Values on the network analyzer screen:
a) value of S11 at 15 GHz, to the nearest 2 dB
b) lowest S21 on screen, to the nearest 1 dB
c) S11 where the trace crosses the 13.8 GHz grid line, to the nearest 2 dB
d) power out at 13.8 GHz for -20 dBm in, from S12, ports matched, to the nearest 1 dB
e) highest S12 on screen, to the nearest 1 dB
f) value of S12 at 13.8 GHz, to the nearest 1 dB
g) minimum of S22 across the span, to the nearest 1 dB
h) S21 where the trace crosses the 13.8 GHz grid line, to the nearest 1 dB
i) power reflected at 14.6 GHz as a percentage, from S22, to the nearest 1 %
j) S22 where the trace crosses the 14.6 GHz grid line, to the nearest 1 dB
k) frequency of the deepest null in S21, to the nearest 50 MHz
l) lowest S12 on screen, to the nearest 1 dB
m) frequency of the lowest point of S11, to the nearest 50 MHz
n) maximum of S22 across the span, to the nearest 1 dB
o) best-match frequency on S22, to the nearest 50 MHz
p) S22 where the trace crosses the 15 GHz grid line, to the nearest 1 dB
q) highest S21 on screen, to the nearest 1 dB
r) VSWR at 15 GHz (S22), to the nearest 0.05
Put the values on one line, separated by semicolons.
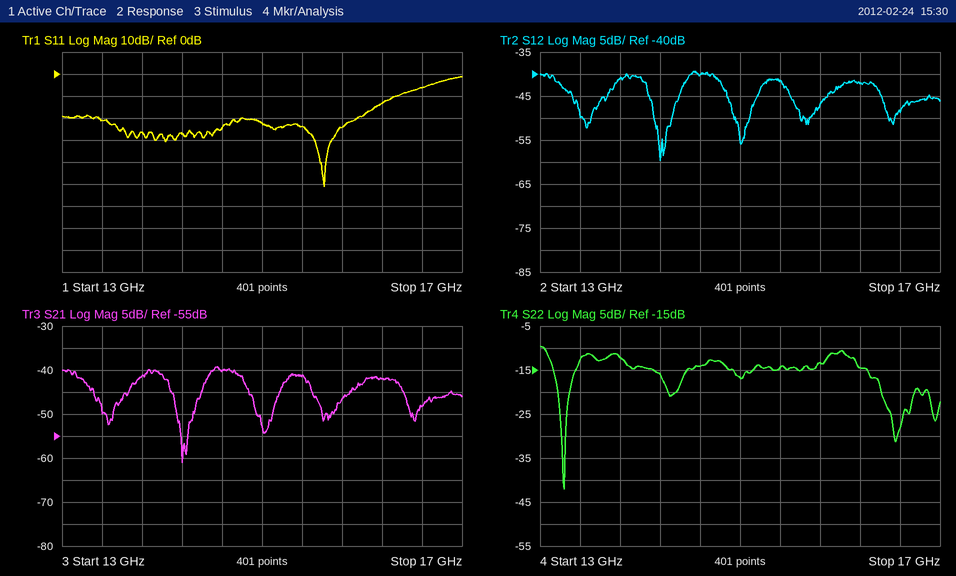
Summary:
-22 dB; -61 dB; -26 dB; -61 dBm; -39 dB; -41 dB; -42 dB; -41 dB; 4 %; -14 dB; 14.20 GHz; -60 dB; 15.60 GHz; -10 dB; 13.25 GHz; -17 dB; -39 dB; 1.35
